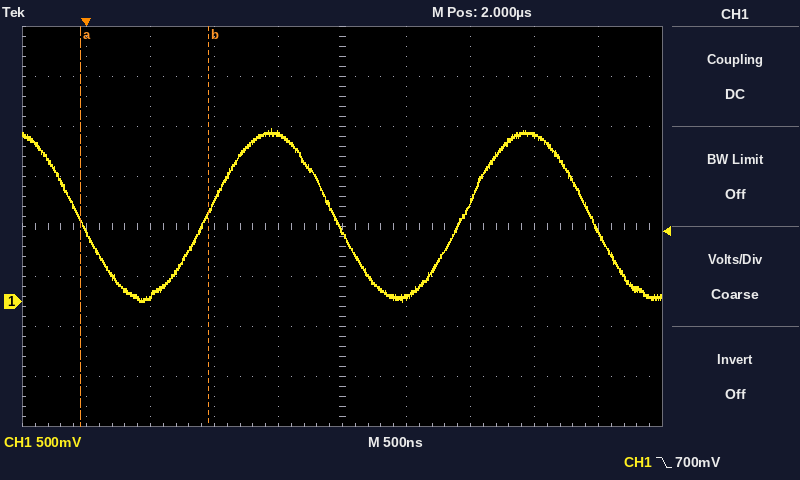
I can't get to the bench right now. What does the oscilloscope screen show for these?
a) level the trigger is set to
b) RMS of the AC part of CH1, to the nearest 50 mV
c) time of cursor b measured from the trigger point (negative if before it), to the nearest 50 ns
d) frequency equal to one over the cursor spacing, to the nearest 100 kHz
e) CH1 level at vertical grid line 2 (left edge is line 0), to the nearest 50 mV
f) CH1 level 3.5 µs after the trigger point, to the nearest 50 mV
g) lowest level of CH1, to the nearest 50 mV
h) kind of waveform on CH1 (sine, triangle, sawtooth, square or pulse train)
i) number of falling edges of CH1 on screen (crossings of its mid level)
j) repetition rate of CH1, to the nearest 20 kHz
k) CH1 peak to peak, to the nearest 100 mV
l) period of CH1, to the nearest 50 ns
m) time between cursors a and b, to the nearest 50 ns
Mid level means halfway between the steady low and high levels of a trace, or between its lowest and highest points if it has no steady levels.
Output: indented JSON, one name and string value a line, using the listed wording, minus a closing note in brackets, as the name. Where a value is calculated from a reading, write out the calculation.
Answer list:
{
  "level the trigger is set to": "700 mV",
  "RMS of the AC part of CH1, to the nearest 50 mV": "1.70 V / (2√2) ≈ 601 mV, so 600 mV to the nearest 50 mV",
  "time of cursor b measured from the trigger point (negative if before it), to the nearest 50 ns": "+950 ns",
  "frequency equal to one over the cursor spacing, to the nearest 100 kHz": "1 / 1.00 µs ≈ 1.0 MHz",
  "CH1 level at vertical grid line 2 (left edge is line 0), to the nearest 50 mV": "50 mV",
  "CH1 level 3.5 µs after the trigger point, to the nearest 50 mV": "1.65 V",
  "lowest level of CH1, to the nearest 50 mV": "0 mV",
  "kind of waveform on CH1": "sine",
  "number of falling edges of CH1 on screen": "3",
  "repetition rate of CH1, to the nearest 20 kHz": "1 / 2.00 µs ≈ 500 kHz",
  "CH1 peak to peak, to the nearest 100 mV": "1.70 V",
  "period of CH1, to the nearest 50 ns": "2.00 µs",
  "time between cursors a and b, to the nearest 50 ns": "1.00 µs"
}
